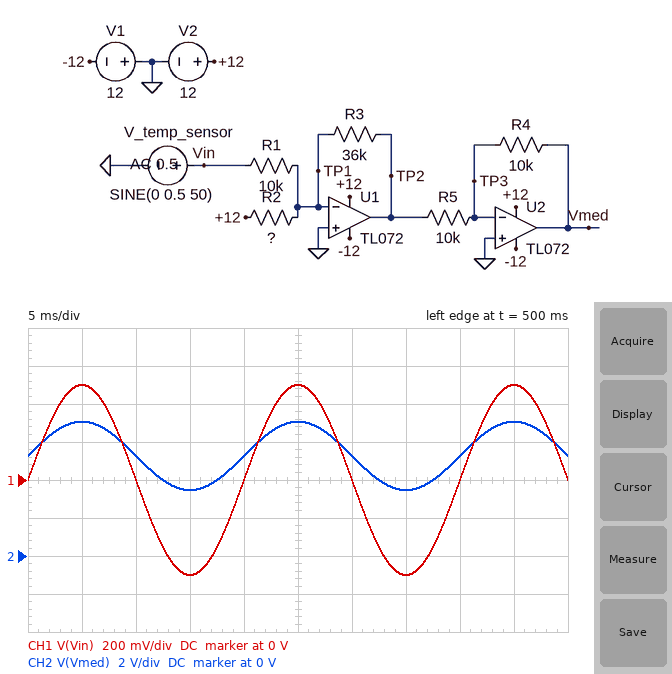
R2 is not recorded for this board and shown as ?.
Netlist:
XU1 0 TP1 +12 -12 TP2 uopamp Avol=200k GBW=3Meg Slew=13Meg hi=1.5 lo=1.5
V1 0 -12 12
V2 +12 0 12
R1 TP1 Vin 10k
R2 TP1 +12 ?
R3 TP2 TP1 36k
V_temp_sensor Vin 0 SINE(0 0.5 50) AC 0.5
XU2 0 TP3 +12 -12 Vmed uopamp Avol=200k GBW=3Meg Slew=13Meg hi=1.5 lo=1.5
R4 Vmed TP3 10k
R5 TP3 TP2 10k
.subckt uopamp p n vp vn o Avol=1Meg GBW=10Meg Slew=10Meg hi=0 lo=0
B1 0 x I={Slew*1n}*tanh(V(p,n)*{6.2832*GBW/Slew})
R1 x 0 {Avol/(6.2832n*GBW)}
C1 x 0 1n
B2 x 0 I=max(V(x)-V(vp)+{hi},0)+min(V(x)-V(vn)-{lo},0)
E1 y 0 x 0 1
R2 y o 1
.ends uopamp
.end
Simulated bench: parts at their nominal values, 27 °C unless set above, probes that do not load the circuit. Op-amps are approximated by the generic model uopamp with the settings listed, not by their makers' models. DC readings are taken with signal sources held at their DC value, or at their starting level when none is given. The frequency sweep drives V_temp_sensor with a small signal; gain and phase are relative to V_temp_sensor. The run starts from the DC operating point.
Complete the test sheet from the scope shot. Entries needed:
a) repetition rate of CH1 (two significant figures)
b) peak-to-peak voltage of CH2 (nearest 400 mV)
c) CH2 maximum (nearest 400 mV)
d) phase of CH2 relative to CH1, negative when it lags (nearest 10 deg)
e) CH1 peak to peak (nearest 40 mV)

50 Hz
3.6 V
7.2 V
0 deg
1.00 V
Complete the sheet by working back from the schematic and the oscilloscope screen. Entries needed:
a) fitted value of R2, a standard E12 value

82 kΩ
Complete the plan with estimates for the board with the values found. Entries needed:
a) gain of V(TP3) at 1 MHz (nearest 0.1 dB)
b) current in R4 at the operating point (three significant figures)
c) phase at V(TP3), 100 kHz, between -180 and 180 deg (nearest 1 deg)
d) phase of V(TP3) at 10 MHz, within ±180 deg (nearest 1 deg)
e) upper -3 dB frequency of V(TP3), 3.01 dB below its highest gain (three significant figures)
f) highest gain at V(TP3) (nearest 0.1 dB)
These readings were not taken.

-5.8 dB
527 µA
-103 deg
102 deg
2.46 MHz
-5.8 dB
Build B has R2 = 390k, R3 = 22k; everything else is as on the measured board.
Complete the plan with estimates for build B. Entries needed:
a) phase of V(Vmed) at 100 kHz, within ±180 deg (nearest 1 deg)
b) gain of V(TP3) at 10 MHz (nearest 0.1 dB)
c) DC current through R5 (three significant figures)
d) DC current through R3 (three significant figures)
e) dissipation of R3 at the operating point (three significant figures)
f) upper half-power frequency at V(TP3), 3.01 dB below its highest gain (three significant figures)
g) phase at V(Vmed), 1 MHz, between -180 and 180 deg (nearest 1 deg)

-10 deg
-20.0 dB
67.7 µA
30.8 µA
20.8 µW
2.90 MHz
-81 deg
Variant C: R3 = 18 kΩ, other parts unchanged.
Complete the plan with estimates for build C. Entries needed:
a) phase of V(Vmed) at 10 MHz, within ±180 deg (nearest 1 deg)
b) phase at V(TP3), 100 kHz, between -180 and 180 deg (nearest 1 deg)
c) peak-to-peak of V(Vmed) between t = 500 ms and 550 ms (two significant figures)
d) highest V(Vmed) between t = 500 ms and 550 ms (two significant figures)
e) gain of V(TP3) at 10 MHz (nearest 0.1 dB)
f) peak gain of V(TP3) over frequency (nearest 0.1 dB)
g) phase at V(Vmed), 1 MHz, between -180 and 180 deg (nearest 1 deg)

-166 deg
-100 deg
1.8 V
3.5 V
-21.1 dB
-8.9 dB
-79 deg
